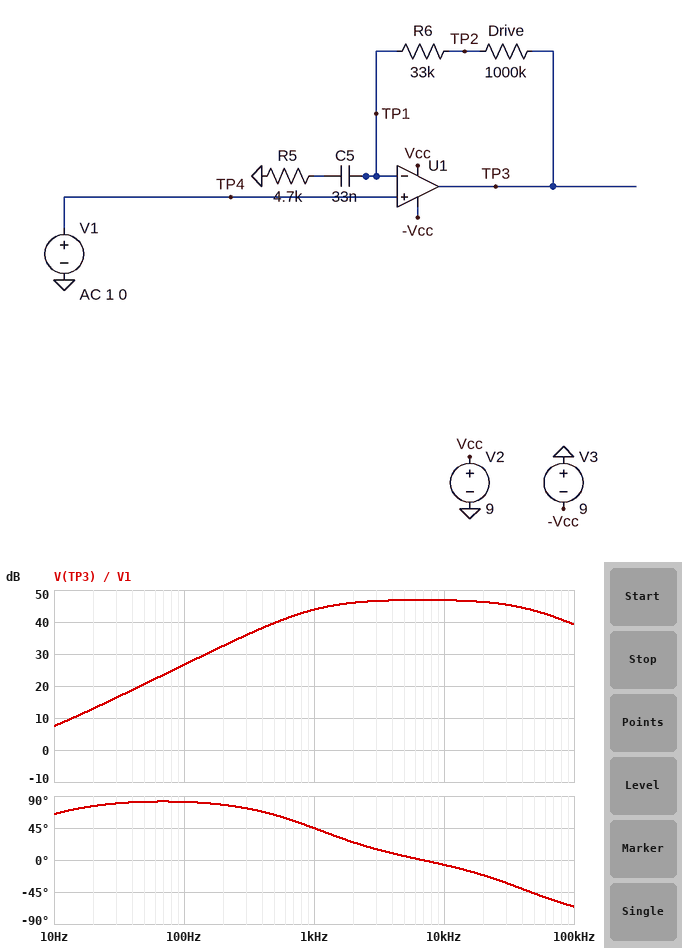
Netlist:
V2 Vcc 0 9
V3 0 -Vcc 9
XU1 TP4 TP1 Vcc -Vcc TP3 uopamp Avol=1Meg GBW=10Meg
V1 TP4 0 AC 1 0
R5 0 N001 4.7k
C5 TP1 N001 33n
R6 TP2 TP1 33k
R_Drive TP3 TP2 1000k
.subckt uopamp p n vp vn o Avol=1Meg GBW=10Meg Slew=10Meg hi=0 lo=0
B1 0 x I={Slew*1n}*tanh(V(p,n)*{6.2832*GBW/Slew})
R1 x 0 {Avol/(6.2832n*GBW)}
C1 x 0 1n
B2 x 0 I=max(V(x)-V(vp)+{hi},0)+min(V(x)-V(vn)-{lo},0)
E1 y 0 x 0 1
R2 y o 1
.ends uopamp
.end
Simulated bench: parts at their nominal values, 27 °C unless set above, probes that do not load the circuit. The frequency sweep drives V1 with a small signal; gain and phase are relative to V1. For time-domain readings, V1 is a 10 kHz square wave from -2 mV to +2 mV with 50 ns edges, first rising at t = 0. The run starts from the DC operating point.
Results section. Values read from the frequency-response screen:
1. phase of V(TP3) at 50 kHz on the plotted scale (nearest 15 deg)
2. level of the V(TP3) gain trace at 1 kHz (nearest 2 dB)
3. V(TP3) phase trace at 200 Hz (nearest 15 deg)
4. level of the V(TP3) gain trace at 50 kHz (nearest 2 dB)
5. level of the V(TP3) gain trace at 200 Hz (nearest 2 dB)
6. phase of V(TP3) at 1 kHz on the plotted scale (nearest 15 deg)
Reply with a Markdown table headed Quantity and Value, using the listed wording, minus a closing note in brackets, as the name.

| Quantity | Value |
|---|---|
| phase of V(TP3) at 50 kHz on the plotted scale | -45 deg |
| level of the V(TP3) gain trace at 1 kHz | 44 dB |
| V(TP3) phase trace at 200 Hz | 75 deg |
| level of the V(TP3) gain trace at 50 kHz | 44 dB |
| level of the V(TP3) gain trace at 200 Hz | 32 dB |
| phase of V(TP3) at 1 kHz on the plotted scale | 45 deg |
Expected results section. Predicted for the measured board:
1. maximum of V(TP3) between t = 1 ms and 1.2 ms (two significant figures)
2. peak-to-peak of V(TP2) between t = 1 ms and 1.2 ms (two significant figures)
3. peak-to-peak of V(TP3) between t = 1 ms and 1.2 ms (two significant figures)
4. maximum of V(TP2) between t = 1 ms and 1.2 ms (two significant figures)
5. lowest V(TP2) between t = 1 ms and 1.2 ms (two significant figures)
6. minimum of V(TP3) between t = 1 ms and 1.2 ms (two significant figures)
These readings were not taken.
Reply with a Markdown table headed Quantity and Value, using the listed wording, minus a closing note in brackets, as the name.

| Quantity | Value |
|---|---|
| maximum of V(TP3) between t = 1 ms and 1.2 ms | 470 mV |
| peak-to-peak of V(TP2) between t = 1 ms and 1.2 ms | 34 mV |
| peak-to-peak of V(TP3) between t = 1 ms and 1.2 ms | 950 mV |
| maximum of V(TP2) between t = 1 ms and 1.2 ms | 17 mV |
| lowest V(TP2) between t = 1 ms and 1.2 ms | -17 mV |
| minimum of V(TP3) between t = 1 ms and 1.2 ms | -470 mV |
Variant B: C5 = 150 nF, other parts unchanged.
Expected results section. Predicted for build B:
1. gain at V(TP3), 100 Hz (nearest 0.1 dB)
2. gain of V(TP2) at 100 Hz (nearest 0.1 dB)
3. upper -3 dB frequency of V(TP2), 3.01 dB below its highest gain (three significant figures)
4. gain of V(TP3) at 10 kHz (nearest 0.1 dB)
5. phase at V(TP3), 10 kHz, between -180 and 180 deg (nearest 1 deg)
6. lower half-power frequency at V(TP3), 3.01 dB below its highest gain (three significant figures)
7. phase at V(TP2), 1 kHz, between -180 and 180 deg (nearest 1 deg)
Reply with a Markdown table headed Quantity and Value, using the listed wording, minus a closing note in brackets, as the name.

| Quantity | Value |
|---|---|
| gain at V(TP3), 100 Hz | 39.0 dB |
| gain of V(TP2) at 100 Hz | 10.6 dB |
| upper -3 dB frequency of V(TP2), 3.01 dB below its highest gain | 45.5 kHz |
| gain of V(TP3) at 10 kHz | 46.7 dB |
| phase at V(TP3), 10 kHz, between -180 and 180 deg | -11 deg |
| lower half-power frequency at V(TP3), 3.01 dB below its highest gain | 225 Hz |
| phase at V(TP2), 1 kHz, between -180 and 180 deg | 10 deg |
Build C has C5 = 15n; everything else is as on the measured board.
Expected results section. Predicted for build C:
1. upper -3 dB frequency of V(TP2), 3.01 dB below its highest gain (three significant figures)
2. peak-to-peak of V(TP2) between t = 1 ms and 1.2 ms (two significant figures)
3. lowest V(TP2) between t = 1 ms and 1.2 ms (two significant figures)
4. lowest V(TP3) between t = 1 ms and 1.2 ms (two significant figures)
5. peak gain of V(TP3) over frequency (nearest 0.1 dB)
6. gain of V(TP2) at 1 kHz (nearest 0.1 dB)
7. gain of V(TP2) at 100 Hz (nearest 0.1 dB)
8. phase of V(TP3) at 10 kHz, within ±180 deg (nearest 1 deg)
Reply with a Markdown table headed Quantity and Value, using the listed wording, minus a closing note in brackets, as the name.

| Quantity | Value |
|---|---|
| upper -3 dB frequency of V(TP2), 3.01 dB below its highest gain | 47.4 kHz |
| peak-to-peak of V(TP2) between t = 1 ms and 1.2 ms | 37 mV |
| lowest V(TP2) between t = 1 ms and 1.2 ms | -19 mV |
| lowest V(TP3) between t = 1 ms and 1.2 ms | -520 mV |
| peak gain of V(TP3) over frequency | 46.9 dB |
| gain of V(TP2) at 1 kHz | 10.6 dB |
| gain of V(TP2) at 100 Hz | 0.5 dB |
| phase of V(TP3) at 10 kHz, within ±180 deg | 0 deg |
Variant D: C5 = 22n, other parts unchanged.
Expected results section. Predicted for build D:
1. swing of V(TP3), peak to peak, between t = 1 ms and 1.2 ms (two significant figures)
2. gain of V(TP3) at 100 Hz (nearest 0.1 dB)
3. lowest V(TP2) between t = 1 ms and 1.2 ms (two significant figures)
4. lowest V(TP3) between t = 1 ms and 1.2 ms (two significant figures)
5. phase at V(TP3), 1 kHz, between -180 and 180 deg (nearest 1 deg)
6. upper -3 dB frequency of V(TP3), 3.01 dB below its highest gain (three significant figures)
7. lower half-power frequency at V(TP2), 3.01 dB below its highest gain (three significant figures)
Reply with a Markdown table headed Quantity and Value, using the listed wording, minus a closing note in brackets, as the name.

| Quantity | Value |
|---|---|
| swing of V(TP3), peak to peak, between t = 1 ms and 1.2 ms | 990 mV |
| gain of V(TP3) at 100 Hz | 23.1 dB |
| lowest V(TP2) between t = 1 ms and 1.2 ms | -18 mV |
| lowest V(TP3) between t = 1 ms and 1.2 ms | -490 mV |
| phase at V(TP3), 1 kHz, between -180 and 180 deg | 56 deg |
| upper -3 dB frequency of V(TP3), 3.01 dB below its highest gain | 46.8 kHz |
| lower half-power frequency at V(TP2), 3.01 dB below its highest gain | 1.47 kHz |
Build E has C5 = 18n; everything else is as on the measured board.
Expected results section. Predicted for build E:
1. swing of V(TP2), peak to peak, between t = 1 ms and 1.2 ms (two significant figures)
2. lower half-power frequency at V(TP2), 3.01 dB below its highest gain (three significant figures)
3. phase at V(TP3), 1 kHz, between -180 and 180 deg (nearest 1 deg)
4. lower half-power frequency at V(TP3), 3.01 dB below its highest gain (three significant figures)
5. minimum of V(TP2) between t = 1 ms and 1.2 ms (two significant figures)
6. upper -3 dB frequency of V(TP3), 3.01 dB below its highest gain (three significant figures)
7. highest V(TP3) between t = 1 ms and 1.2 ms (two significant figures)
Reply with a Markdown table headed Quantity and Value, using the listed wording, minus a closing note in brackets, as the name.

| Quantity | Value |
|---|---|
| swing of V(TP2), peak to peak, between t = 1 ms and 1.2 ms | 36 mV |
| lower half-power frequency at V(TP2), 3.01 dB below its highest gain | 1.78 kHz |
| phase at V(TP3), 1 kHz, between -180 and 180 deg | 61 deg |
| lower half-power frequency at V(TP3), 3.01 dB below its highest gain | 1.81 kHz |
| minimum of V(TP2) between t = 1 ms and 1.2 ms | -18 mV |
| upper -3 dB frequency of V(TP3), 3.01 dB below its highest gain | 47.1 kHz |
| highest V(TP3) between t = 1 ms and 1.2 ms | 510 mV |
